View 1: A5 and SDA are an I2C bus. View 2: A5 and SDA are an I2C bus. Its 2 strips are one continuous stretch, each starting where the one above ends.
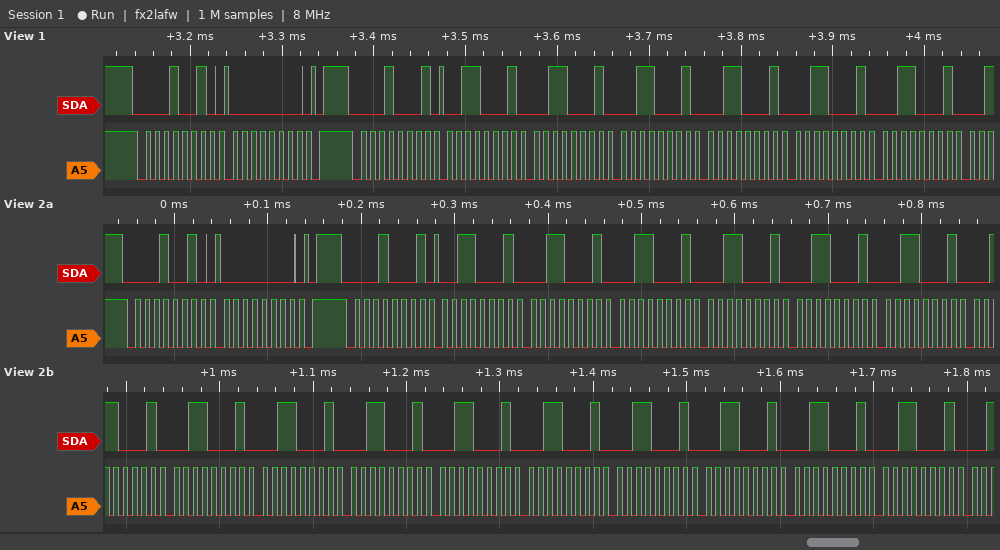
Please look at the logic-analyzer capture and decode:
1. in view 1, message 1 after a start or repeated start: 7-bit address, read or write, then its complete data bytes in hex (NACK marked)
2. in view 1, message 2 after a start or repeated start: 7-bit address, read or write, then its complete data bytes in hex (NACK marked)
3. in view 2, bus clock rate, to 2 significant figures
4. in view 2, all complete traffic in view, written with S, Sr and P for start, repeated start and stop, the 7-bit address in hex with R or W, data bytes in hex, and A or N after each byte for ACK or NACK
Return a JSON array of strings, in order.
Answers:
["0x09 write: 00", "0x08 read: 31 31 31 31 31 31", "100 kHz", "S 09W A 00 A P S 08R A 31 A 31 A 31 A 31 A 31 A 31 A 31 A 31 A 31 A 31 A 31 A 31 A 31 A 31 A 31 A 31 A"]
